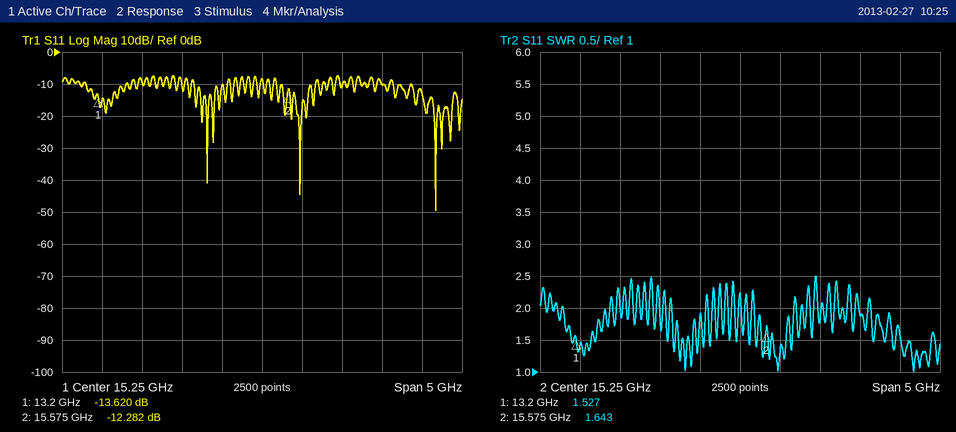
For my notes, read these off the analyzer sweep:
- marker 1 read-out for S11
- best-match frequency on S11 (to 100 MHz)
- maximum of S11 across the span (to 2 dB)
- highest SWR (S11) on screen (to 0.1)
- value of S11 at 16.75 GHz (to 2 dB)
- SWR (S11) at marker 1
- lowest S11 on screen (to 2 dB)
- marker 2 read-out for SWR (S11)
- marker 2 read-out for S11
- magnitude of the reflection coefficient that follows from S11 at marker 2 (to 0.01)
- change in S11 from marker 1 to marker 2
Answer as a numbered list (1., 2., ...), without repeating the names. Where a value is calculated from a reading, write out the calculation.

1. -13.620 dB
2. 17.4 GHz
3. -8 dB
4. 2.5
5. -10 dB
6. 1.527
7. -50 dB
8. 1.643
9. -12.282 dB
10. 10^(-12.282/20) ≈ 0.24
11. -12.282 − (-13.62) = 1.338 dB
